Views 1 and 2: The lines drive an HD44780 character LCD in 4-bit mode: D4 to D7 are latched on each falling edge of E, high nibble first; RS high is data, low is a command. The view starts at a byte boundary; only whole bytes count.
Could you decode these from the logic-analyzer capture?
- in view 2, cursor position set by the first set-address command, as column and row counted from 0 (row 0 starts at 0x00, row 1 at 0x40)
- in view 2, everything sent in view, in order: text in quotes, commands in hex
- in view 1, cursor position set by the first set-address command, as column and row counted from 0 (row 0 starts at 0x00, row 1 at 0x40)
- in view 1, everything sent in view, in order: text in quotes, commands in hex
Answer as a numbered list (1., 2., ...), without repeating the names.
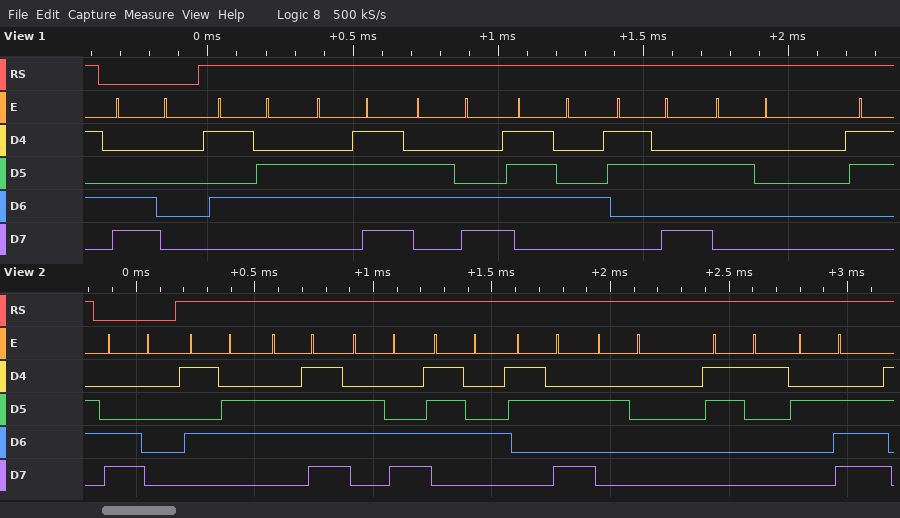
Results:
1. column 0, row 1
2. 0xC0 "Volt: 1."
3. column 0, row 1
4. 0xC0 "Volt: "
